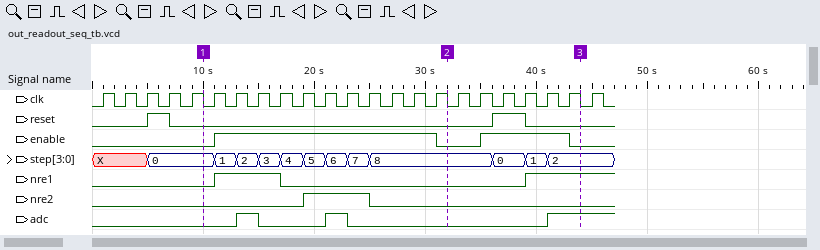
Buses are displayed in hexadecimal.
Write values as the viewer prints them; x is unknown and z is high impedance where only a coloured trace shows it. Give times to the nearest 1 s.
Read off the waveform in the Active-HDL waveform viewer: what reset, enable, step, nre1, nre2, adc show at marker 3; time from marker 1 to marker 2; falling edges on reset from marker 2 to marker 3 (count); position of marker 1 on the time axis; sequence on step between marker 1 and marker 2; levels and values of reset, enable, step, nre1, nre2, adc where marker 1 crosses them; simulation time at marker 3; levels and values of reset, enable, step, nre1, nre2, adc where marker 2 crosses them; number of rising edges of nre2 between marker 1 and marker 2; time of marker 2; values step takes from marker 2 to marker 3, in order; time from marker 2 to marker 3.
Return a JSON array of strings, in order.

["reset=0, enable=0, step=2, nre1=1, nre2=0, adc=1", "22 s", "1", "10 s", "0, 1, 2, 3, 4, 5, 6, 7, 8", "reset=0, enable=0, step=0, nre1=0, nre2=0, adc=0", "44 s", "reset=0, enable=0, step=8, nre1=0, nre2=0, adc=0", "1", "32 s", "8, 0, 1, 2", "12 s"]
